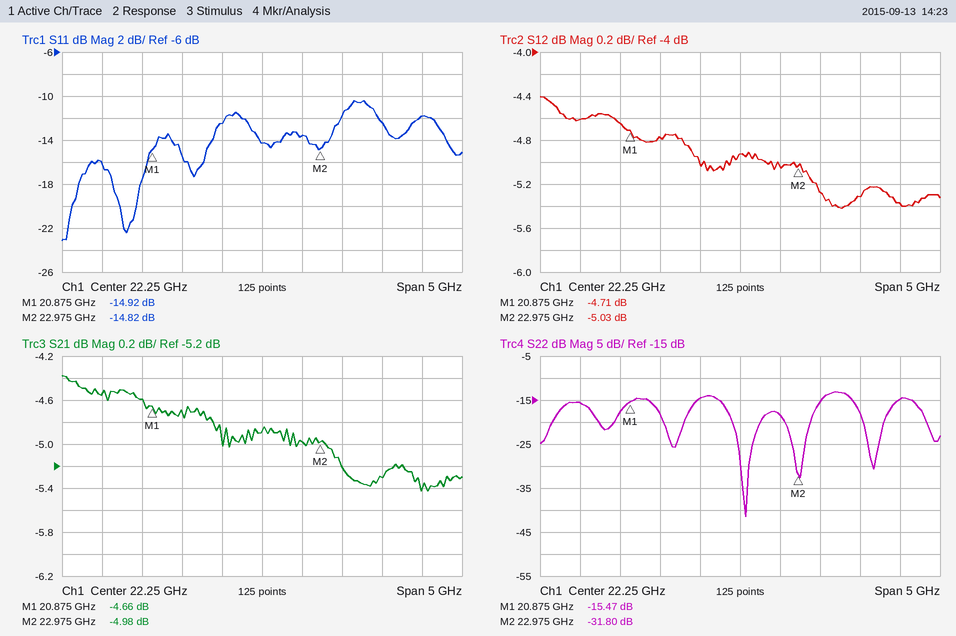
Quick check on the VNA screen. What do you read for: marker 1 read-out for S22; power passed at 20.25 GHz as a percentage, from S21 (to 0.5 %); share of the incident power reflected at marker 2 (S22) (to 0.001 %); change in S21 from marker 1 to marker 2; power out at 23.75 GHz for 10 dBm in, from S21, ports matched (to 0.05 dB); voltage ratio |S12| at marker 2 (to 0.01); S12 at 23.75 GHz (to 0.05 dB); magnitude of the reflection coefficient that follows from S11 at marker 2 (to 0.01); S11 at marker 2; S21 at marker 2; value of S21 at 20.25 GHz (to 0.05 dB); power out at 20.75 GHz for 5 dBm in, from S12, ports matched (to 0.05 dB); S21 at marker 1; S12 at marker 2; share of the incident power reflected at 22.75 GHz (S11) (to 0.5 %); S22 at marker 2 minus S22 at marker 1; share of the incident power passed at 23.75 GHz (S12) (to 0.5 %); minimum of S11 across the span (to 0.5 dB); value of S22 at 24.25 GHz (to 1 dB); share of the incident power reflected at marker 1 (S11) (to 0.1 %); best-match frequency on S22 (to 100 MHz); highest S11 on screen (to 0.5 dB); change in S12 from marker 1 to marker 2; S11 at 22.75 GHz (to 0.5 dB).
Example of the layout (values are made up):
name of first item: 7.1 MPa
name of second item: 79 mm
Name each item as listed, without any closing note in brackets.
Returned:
marker 1 read-out for S22: -15.47 dB
power passed at 20.25 GHz as a percentage, from S21: 35.0 %
share of the incident power reflected at marker 2 (S22): 0.066 %
change in S21 from marker 1 to marker 2: -0.32 dB
power out at 23.75 GHz for 10 dBm in, from S21, ports matched: 4.70 dBm
voltage ratio |S12| at marker 2: 0.56
S12 at 23.75 GHz: -5.30 dB
magnitude of the reflection coefficient that follows from S11 at marker 2: 0.18
S11 at marker 2: -14.82 dB
S21 at marker 2: -4.98 dB
value of S21 at 20.25 GHz: -4.55 dB
power out at 20.75 GHz for 5 dBm in, from S12, ports matched: 0.35 dBm
S21 at marker 1: -4.66 dB
S12 at marker 2: -5.03 dB
share of the incident power reflected at 22.75 GHz (S11): 4.5 %
S22 at marker 2 minus S22 at marker 1: -16.33 dB
share of the incident power passed at 23.75 GHz (S12): 29.5 %
minimum of S11 across the span: -23.0 dB
value of S22 at 24.25 GHz: -15 dB
share of the incident power reflected at marker 1 (S11): 3.2 %
best-match frequency on S22: 22.3 GHz
highest S11 on screen: -10.5 dB
change in S12 from marker 1 to marker 2: -0.32 dB
S11 at 22.75 GHz: -13.5 dB
